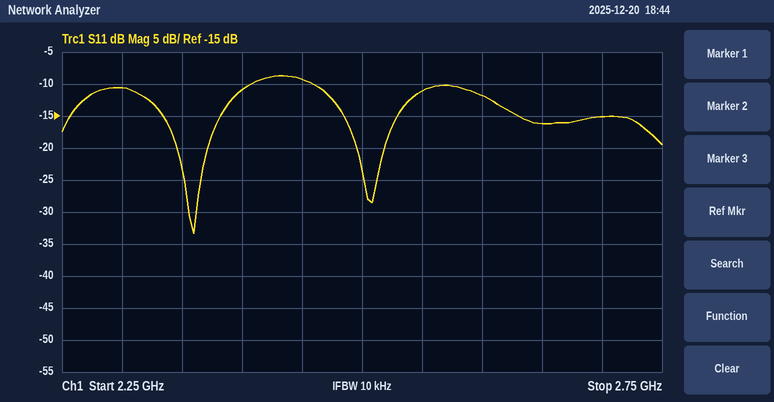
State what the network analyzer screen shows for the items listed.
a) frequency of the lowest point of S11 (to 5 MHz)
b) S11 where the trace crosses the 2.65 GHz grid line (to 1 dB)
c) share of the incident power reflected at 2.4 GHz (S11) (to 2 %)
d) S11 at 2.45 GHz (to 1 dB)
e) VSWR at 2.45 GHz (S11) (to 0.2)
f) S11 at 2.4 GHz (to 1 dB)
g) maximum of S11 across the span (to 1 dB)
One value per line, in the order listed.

2.360 GHz
-16 dB
8 %
-9 dB
2.0
-11 dB
-9 dB
